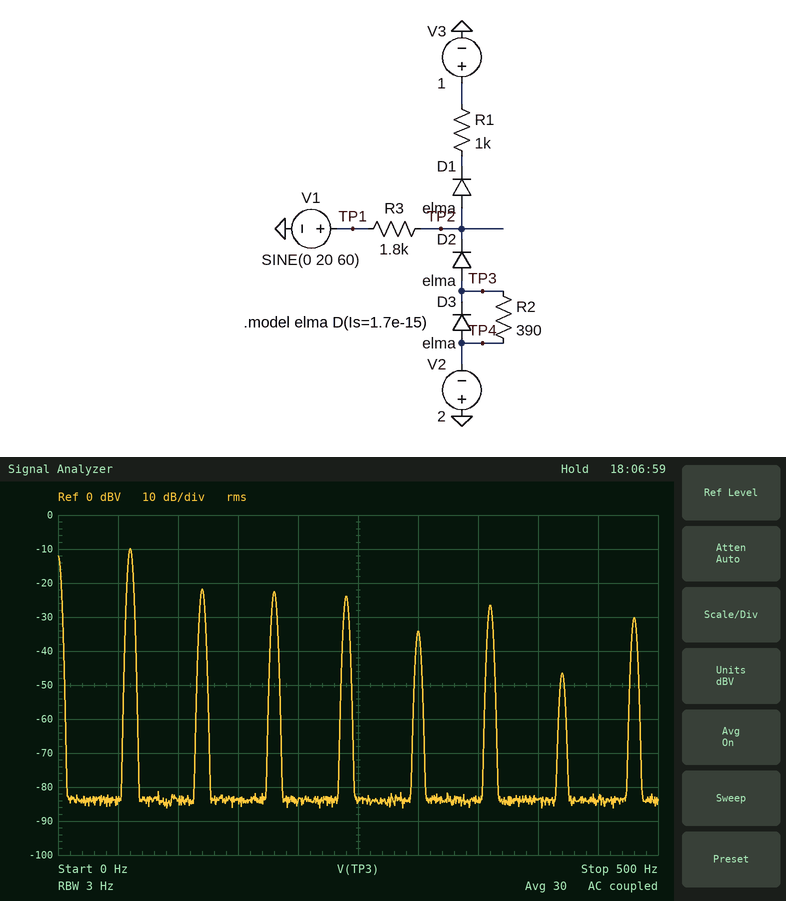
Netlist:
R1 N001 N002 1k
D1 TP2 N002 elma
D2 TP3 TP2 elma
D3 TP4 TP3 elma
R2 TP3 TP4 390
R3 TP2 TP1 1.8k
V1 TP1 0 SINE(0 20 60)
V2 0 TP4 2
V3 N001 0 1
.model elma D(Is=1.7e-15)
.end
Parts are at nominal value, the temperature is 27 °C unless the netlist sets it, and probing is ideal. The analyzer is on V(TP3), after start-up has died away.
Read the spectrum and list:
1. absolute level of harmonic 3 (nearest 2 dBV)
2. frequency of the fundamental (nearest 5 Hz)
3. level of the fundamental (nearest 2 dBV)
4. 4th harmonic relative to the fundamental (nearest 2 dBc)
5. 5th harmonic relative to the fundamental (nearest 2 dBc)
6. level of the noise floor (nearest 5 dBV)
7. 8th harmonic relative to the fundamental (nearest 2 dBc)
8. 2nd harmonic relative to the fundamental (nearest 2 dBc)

-22 dBV
60 Hz
-10 dBV
-14 dBc
-24 dBc
-85 dBV
-20 dBc
-12 dBc
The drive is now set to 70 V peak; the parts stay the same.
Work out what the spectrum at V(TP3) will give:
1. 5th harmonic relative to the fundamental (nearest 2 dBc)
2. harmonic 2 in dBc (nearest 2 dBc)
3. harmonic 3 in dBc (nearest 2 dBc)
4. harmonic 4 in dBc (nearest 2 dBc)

-16 dBc
-20 dBc
-10 dBc
-22 dBc
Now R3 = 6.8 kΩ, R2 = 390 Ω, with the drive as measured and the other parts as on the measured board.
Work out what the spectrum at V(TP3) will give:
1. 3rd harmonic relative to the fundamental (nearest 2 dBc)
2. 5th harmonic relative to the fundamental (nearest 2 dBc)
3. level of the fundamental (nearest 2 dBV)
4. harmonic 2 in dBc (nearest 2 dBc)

-28 dBc
-22 dBc
-12 dBV
-8 dBc
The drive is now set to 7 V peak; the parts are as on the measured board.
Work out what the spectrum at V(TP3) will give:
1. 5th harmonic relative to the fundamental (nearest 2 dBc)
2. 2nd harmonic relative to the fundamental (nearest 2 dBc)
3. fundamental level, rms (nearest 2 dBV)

-18 dBc
-4 dBc
-14 dBV
